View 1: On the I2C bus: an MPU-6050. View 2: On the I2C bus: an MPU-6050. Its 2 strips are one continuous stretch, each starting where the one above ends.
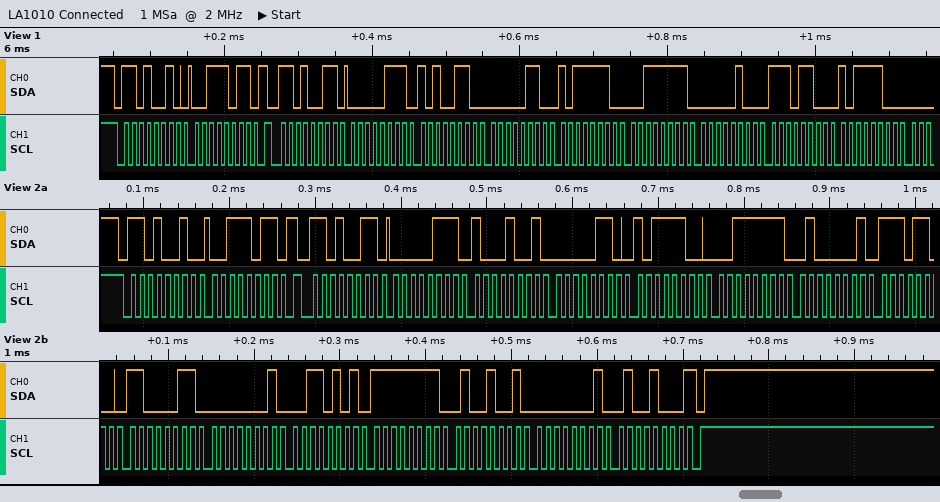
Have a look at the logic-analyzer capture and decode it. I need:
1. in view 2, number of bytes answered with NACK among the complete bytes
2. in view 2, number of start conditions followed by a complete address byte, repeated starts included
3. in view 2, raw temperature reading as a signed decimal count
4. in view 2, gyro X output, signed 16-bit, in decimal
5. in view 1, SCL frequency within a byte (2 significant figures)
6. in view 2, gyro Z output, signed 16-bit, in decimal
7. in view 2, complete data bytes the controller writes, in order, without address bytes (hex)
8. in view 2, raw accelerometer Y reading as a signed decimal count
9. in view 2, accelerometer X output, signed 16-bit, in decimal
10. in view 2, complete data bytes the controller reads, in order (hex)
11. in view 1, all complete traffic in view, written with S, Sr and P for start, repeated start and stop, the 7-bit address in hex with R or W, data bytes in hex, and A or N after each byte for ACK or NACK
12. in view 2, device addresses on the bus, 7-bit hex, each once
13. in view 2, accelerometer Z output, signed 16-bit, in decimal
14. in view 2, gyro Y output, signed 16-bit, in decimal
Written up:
1
2
-4925
309
100 kHz
328
3B
1724
1929
07 89 06 BC 3F 41 EC C3 01 35 FF 49 01 48
S 69W A 3B A Sr 69R A 07 A A6 A 06 A BE A 3F A 04 A EC A BC A
0x69
16193
-183
